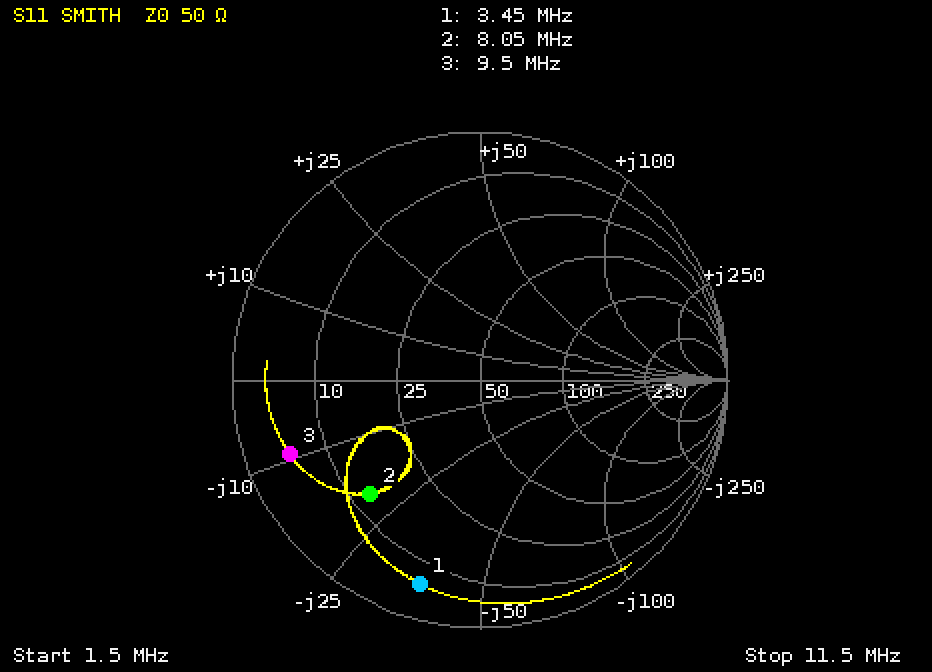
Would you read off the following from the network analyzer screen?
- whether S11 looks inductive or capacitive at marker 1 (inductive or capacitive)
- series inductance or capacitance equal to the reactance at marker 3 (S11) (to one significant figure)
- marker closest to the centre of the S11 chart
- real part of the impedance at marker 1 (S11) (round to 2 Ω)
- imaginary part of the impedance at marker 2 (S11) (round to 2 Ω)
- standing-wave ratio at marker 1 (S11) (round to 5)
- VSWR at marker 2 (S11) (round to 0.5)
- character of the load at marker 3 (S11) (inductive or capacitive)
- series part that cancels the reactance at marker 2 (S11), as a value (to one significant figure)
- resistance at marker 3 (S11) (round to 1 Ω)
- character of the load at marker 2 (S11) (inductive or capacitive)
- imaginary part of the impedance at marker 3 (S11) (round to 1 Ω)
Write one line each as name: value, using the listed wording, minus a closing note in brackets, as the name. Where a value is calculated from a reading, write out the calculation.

whether S11 looks inductive or capacitive at marker 1: capacitive
series inductance or capacitance equal to the reactance at marker 3 (S11): C = 1/(2π × 9.5 MHz × 9 Ω) ≈ 2 nF
marker closest to the centre of the S11 chart: marker 2
real part of the impedance at marker 1 (S11): 6 Ω
imaginary part of the impedance at marker 2 (S11): -20 Ω
standing-wave ratio at marker 1 (S11): 15
VSWR at marker 2 (S11): 4.5
character of the load at marker 3 (S11): capacitive
series part that cancels the reactance at marker 2 (S11), as a value: L = 20 Ω/(2π × 8.05 MHz) ≈ 395 nH, so 400 nH to one significant figure
resistance at marker 3 (S11): 5 Ω
character of the load at marker 2 (S11): capacitive
imaginary part of the impedance at marker 3 (S11): -9 Ω
